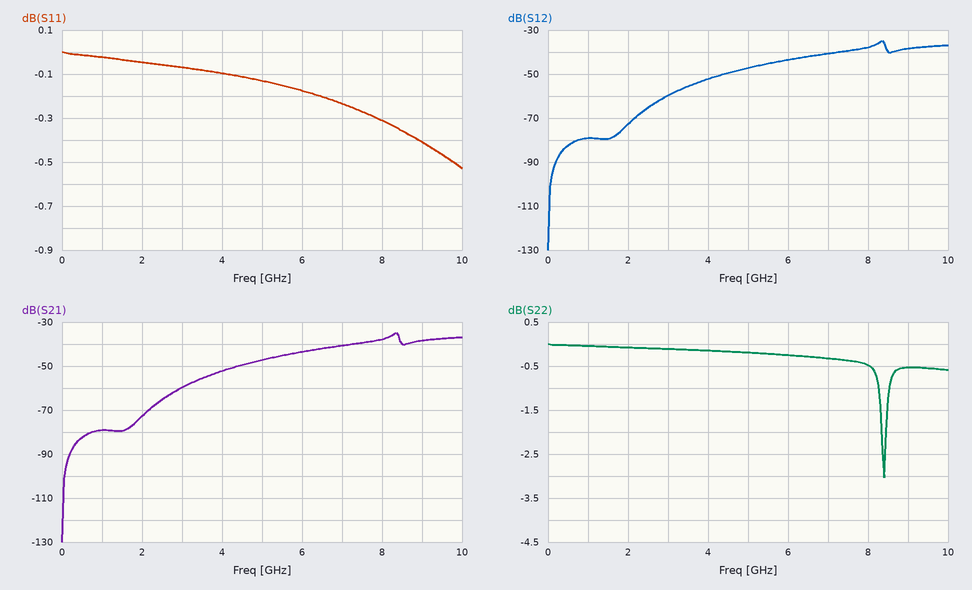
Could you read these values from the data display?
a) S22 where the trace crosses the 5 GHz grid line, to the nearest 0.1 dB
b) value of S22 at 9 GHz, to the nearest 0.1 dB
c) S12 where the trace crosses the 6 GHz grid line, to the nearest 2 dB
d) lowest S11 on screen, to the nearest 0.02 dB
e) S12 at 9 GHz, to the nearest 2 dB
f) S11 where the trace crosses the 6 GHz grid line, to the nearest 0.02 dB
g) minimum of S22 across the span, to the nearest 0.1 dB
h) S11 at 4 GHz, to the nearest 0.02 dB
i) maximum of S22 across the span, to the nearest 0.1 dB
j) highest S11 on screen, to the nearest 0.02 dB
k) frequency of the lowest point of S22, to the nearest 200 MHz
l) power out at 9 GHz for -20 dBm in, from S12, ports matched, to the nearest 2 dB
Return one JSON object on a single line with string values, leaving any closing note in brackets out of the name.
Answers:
{"S22 where the trace crosses the 5 GHz grid line, to the nearest 0.1 dB": "-0.2 dB", "value of S22 at 9 GHz, to the nearest 0.1 dB": "-0.5 dB", "S12 where the trace crosses the 6 GHz grid line, to the nearest 2 dB": "-44 dB", "lowest S11 on screen, to the nearest 0.02 dB": "-0.52 dB", "S12 at 9 GHz, to the nearest 2 dB": "-38 dB", "S11 where the trace crosses the 6 GHz grid line, to the nearest 0.02 dB": "-0.18 dB", "minimum of S22 across the span, to the nearest 0.1 dB": "-3.0 dB", "S11 at 4 GHz, to the nearest 0.02 dB": "-0.10 dB", "maximum of S22 across the span, to the nearest 0.1 dB": "0.0 dB", "highest S11 on screen, to the nearest 0.02 dB": "0.00 dB", "frequency of the lowest point of S22, to the nearest 200 MHz": "8.4 GHz", "power out at 9 GHz for -20 dBm in, from S12, ports matched, to the nearest 2 dB": "-58 dBm"}
